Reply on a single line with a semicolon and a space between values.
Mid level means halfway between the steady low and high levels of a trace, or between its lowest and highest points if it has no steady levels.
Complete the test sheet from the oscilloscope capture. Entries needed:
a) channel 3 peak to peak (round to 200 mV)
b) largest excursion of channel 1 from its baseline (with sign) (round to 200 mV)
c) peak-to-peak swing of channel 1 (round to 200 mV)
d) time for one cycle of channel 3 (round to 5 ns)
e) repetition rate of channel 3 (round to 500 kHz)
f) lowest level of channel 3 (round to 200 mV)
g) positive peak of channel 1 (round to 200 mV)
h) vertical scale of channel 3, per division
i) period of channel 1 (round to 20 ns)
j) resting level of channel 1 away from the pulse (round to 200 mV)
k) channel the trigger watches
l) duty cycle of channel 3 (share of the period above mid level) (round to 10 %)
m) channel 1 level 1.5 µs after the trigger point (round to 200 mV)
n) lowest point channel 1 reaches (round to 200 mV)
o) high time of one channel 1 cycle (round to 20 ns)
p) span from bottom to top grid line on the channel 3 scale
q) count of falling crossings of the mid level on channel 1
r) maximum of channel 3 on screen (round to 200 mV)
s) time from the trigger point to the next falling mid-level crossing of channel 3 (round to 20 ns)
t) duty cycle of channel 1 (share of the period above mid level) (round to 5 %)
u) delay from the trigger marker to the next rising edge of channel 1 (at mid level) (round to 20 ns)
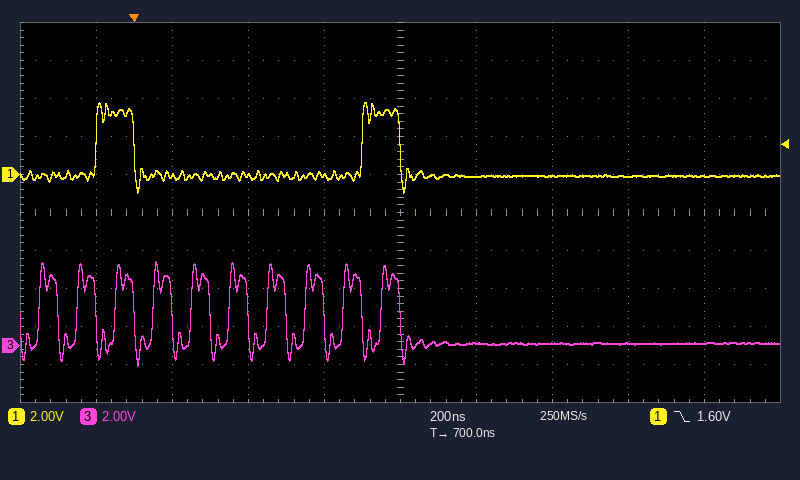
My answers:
5.4 V; +3.8 V; 4.8 V; 100 ns; 10.0 MHz; -1.0 V; 3.8 V; 2 V; 700 ns; 0.0 V; channel 1; 50 %; 0.0 V; -1.0 V; 100 ns; 20 V; 2; 4.4 V; 100 ns; 15 %; 600 ns
